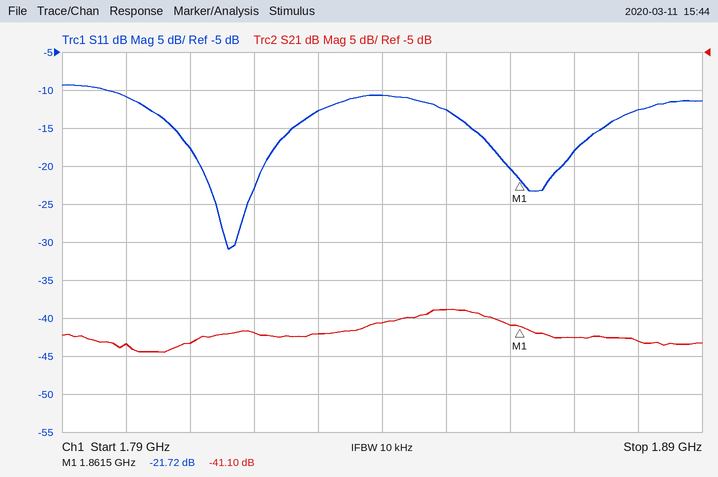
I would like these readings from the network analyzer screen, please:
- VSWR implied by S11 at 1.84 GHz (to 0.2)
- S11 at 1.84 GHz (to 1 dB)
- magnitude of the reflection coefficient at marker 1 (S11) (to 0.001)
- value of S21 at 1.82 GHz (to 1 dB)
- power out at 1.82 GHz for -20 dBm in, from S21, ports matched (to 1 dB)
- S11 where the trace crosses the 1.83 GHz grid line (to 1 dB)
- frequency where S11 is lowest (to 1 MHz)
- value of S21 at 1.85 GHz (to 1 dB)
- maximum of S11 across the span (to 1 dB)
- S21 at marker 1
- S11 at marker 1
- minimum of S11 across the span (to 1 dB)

1.8
-11 dB
0.082
-42 dB
-62 dBm
-13 dB
1.816 GHz
-39 dB
-9 dB
-41.10 dB
-21.72 dB
-31 dB
